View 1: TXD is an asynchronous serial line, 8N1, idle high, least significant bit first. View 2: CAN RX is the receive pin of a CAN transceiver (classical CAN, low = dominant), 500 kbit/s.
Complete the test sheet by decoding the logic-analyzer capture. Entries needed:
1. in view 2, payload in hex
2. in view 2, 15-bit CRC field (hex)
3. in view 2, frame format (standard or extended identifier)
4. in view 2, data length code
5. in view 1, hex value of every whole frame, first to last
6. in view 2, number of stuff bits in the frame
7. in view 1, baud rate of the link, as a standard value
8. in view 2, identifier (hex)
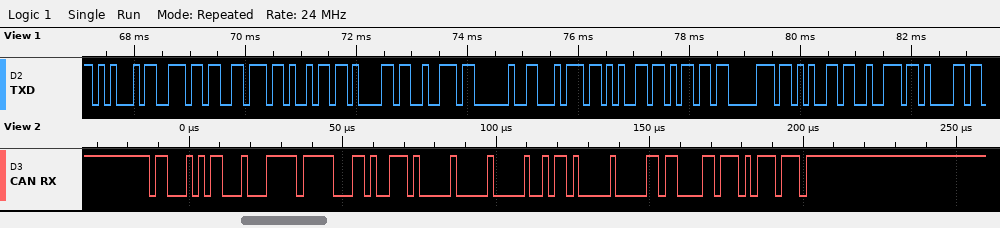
FF CD 3A 00 00 B4 00 B0
0x6EBB
standard
8
45 6E 76 69 61 72 20 74 65 6D 70 65 72 61
7
9600 baud
0x62B
